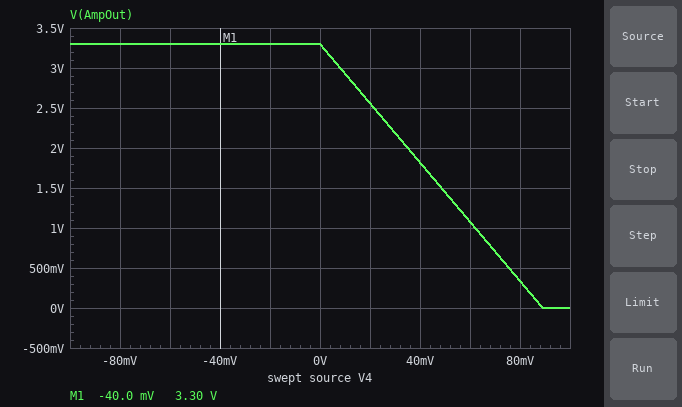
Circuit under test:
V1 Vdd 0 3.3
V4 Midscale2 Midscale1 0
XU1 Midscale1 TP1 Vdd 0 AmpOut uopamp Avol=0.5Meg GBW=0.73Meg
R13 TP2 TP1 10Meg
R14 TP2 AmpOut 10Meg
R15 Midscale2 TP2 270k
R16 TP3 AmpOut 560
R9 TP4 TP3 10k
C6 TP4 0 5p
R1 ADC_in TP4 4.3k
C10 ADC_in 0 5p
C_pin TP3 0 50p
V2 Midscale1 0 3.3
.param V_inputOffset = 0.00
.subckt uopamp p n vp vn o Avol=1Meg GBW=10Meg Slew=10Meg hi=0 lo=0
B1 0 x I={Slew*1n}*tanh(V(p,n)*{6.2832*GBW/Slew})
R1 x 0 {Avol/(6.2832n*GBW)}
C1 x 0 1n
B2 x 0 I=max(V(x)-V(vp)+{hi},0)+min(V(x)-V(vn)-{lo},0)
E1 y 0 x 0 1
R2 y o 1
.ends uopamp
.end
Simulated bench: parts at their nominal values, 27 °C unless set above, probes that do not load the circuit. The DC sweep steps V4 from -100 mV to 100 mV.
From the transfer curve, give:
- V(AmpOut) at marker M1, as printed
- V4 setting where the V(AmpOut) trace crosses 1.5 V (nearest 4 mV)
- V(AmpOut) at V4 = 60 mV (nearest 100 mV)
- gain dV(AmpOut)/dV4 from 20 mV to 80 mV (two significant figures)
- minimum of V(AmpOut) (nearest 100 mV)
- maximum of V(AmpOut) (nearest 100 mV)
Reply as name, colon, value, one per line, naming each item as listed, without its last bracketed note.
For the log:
V(AmpOut) at marker M1, as printed: 3.30 V
V4 setting where the V(AmpOut) trace crosses 1.5 V: 48 mV
V(AmpOut) at V4 = 60 mV: 1.1 V
gain dV(AmpOut)/dV4 from 20 mV to 80 mV: -37 V/V
minimum of V(AmpOut): 0 V
maximum of V(AmpOut): 3.3 V
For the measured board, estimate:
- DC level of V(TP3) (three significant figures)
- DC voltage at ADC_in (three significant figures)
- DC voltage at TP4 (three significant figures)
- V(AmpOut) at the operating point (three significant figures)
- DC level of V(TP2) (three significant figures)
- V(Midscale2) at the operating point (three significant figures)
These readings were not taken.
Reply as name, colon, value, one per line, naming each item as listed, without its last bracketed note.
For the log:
DC level of V(TP3): 3.30 V
DC voltage at ADC_in: 3.30 V
DC voltage at TP4: 3.30 V
V(AmpOut) at the operating point: 3.30 V
DC level of V(TP2): 3.30 V
V(Midscale2) at the operating point: 3.30 V
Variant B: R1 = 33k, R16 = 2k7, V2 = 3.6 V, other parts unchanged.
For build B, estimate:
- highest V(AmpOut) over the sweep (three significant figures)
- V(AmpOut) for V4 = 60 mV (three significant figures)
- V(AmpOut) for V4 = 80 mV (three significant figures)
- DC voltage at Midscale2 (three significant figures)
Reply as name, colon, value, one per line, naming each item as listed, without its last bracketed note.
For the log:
highest V(AmpOut) over the sweep: 3.30 V
V(AmpOut) for V4 = 60 mV: 1.38 V
V(AmpOut) for V4 = 80 mV: 637 mV
DC voltage at Midscale2: 3.60 V
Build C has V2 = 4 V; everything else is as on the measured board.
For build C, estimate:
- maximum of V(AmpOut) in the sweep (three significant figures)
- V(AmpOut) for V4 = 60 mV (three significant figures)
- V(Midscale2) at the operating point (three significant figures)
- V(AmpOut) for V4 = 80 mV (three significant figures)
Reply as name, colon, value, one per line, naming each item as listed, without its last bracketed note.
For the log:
maximum of V(AmpOut) in the sweep: 3.30 V
V(AmpOut) for V4 = 60 mV: 1.78 V
V(Midscale2) at the operating point: 4.00 V
V(AmpOut) for V4 = 80 mV: 1.04 V
